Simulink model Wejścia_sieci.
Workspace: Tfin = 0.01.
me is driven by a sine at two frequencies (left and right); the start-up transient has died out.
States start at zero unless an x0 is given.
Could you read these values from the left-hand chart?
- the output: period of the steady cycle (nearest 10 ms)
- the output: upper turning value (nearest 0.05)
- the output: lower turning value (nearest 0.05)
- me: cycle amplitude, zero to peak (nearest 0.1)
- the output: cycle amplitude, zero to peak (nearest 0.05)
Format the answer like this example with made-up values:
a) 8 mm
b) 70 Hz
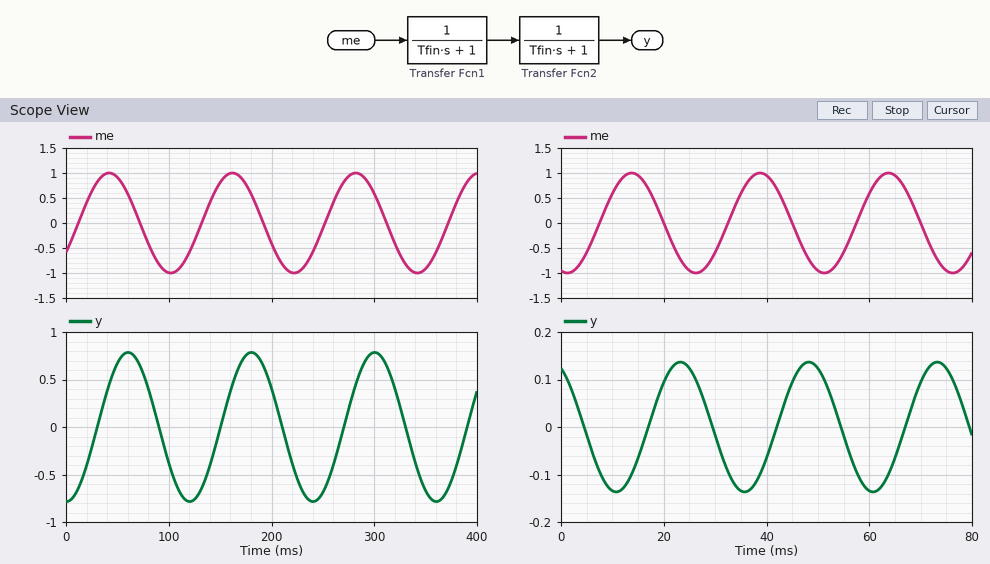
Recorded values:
a) 120 ms
b) 0.80
c) -0.80
d) 1.0
e) 0.80
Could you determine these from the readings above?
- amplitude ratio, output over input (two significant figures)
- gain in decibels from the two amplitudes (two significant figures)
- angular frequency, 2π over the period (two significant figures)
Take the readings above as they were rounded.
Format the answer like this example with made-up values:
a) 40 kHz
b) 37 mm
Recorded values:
a) 0.80
b) -1.9 dB
c) 0.052 rad/ms
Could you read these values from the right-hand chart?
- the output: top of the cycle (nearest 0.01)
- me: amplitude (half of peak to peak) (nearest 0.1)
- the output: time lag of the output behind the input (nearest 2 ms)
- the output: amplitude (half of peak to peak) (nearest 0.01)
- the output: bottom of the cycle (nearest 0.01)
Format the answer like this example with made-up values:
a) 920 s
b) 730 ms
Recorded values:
a) 0.14
b) 1.0
c) 10 ms
d) 0.14
e) -0.14
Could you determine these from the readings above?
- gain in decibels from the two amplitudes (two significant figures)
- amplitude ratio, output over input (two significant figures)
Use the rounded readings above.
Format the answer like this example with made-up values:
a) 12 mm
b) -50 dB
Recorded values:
a) -17 dB
b) 0.14
